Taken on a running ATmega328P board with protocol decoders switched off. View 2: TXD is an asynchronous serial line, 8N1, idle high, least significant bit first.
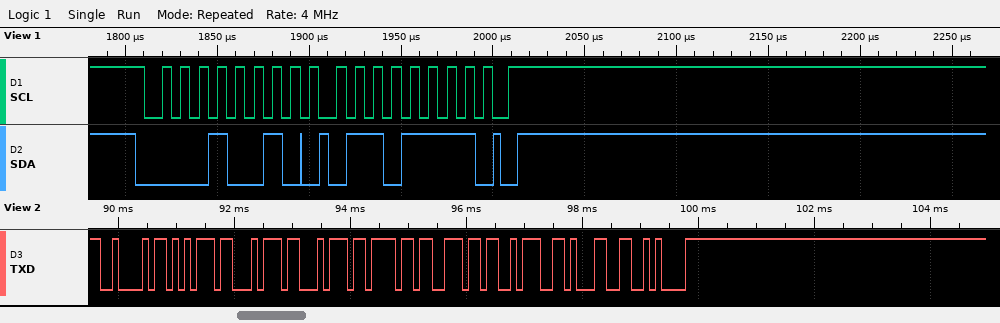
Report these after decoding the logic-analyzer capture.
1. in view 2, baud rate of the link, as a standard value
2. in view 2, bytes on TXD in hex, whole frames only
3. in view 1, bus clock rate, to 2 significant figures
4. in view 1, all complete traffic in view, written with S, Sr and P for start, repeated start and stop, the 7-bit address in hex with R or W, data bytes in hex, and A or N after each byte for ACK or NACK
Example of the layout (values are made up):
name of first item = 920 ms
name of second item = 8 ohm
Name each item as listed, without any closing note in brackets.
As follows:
in view 2, baud rate of the link, as a standard value = 9600 baud
in view 2, bytes on TXD in hex, whole frames only = 42 75 74 74 6F 6E 3A 31 0A
in view 1, bus clock rate, to 2 significant figures = 100 kHz
in view 1, all complete traffic in view, written with S, Sr and P for start, repeated start and stop, the 7-bit address in hex with R or W, data bytes in hex, and A or N after each byte for ACK or NACK = S 09W A 6F A P
